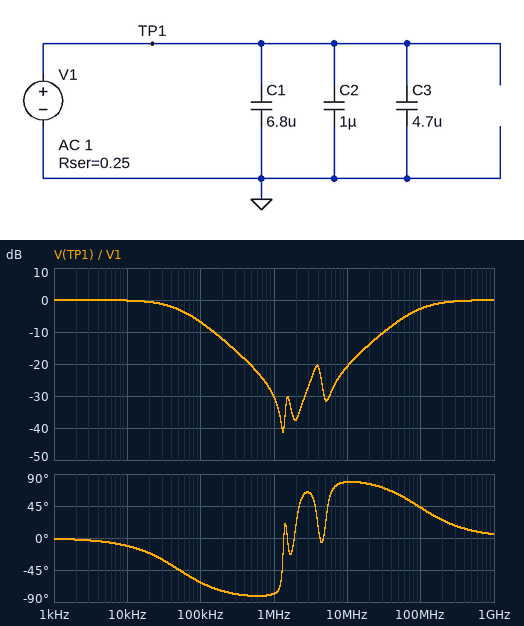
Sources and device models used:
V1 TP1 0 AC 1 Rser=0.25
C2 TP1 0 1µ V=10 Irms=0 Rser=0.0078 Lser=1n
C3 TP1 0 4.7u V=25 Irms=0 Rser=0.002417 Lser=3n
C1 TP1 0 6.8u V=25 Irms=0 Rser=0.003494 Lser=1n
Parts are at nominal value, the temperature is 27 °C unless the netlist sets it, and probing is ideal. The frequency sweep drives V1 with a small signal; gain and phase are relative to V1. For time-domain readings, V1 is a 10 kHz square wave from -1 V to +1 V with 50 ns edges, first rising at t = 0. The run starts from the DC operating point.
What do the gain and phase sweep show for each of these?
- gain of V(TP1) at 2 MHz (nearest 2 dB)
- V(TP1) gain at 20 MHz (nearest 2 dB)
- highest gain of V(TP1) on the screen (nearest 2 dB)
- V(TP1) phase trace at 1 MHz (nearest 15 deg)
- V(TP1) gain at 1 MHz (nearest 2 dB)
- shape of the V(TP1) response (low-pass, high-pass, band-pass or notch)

-38 dB
-14 dB
0 dB
-75 deg
-30 dB
notch
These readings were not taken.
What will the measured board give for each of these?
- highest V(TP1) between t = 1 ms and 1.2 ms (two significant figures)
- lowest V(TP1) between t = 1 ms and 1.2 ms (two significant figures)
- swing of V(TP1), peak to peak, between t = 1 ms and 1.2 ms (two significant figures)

1.0 V
-1.0 V
2.0 V
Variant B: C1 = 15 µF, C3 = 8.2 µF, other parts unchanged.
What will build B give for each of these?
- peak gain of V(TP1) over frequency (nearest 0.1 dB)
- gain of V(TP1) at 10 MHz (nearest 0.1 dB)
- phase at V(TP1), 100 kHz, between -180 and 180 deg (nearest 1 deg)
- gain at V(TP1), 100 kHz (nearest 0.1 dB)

0 dB
-20.6 dB
-74 deg
-12.0 dB
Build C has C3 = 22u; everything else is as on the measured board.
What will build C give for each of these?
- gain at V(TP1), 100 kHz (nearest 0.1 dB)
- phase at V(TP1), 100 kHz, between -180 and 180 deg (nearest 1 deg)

-13.8 dB
-77 deg
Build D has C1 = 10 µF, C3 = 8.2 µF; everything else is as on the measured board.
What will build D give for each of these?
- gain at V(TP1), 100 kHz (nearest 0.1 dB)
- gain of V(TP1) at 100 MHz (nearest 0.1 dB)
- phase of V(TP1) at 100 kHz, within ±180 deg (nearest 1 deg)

-10.1 dB
-2.7 dB
-71 deg
